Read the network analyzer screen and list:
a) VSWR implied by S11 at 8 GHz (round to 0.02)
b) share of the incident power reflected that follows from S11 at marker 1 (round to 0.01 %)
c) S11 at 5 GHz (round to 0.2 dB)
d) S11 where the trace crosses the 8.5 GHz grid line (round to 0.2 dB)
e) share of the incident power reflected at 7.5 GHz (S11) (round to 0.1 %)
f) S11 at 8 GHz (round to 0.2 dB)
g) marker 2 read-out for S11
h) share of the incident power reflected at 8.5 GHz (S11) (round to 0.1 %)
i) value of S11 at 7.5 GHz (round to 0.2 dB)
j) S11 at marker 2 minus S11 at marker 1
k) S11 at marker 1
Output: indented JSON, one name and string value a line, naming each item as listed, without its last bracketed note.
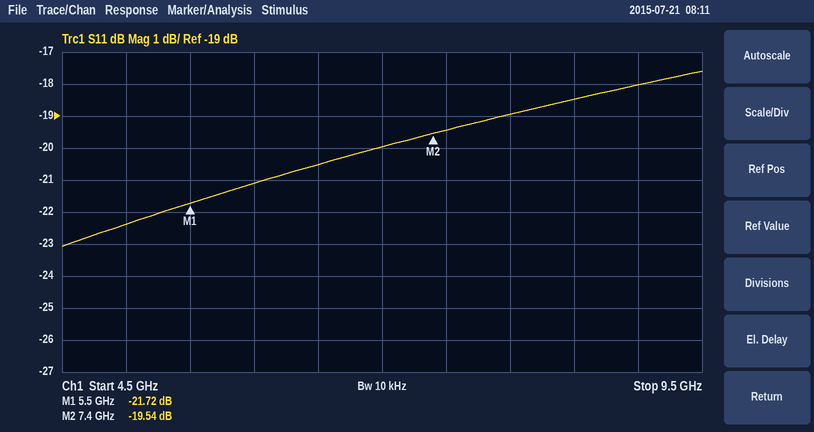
{
  "VSWR implied by S11 at 8 GHz": "1.26",
  "share of the incident power reflected that follows from S11 at marker 1": "0.67 %",
  "S11 at 5 GHz": "-22.4 dB",
  "S11 where the trace crosses the 8.5 GHz grid line": "-18.4 dB",
  "share of the incident power reflected at 7.5 GHz (S11)": "1.1 %",
  "S11 at 8 GHz": "-19.0 dB",
  "marker 2 read-out for S11": "-19.54 dB",
  "share of the incident power reflected at 8.5 GHz (S11)": "1.4 %",
  "value of S11 at 7.5 GHz": "-19.4 dB",
  "S11 at marker 2 minus S11 at marker 1": "2.18 dB",
  "S11 at marker 1": "-21.72 dB"
}
